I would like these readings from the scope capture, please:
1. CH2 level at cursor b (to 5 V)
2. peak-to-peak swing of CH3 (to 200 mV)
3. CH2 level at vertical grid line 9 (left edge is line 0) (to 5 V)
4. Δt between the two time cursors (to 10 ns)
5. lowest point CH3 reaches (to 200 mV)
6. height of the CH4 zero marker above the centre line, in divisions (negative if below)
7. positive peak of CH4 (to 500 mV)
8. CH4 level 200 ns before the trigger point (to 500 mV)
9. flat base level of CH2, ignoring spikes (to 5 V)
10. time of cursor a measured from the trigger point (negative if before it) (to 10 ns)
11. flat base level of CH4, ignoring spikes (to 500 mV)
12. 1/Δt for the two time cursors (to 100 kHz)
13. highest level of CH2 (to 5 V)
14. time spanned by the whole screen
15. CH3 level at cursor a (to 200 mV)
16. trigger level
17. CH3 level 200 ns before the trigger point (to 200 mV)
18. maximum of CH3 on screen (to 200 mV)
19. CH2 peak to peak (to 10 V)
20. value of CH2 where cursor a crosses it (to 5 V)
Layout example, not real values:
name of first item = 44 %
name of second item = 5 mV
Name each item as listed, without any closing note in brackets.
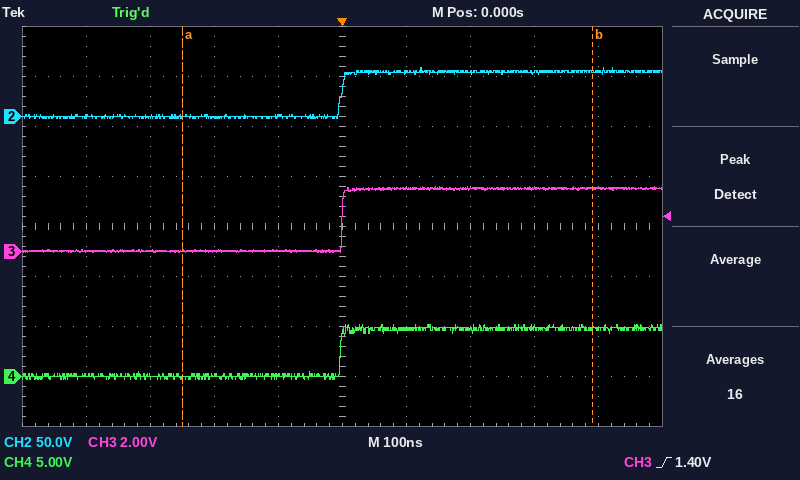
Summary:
CH2 level at cursor b = 45 V
peak-to-peak swing of CH3 = 2.6 V
CH2 level at vertical grid line 9 (left edge is line 0) = 45 V
Δt between the two time cursors = 640 ns
lowest point CH3 reaches = 0.0 V
height of the CH4 zero marker above the centre line, in divisions = -3.0 div
positive peak of CH4 = 5.0 V
CH4 level 200 ns before the trigger point = 0.0 V
flat base level of CH2, ignoring spikes = 0 V
time of cursor a measured from the trigger point (negative if before it) = -250 ns
flat base level of CH4, ignoring spikes = 0.0 V
1/Δt for the two time cursors = 1.6 MHz
highest level of CH2 = 50 V
time spanned by the whole screen = 1 µs
CH3 level at cursor a = 0.0 V
trigger level = 1.40 V
CH3 level 200 ns before the trigger point = 0.0 V
maximum of CH3 on screen = 2.6 V
CH2 peak to peak = 50 V
value of CH2 where cursor a crosses it = 0 V
